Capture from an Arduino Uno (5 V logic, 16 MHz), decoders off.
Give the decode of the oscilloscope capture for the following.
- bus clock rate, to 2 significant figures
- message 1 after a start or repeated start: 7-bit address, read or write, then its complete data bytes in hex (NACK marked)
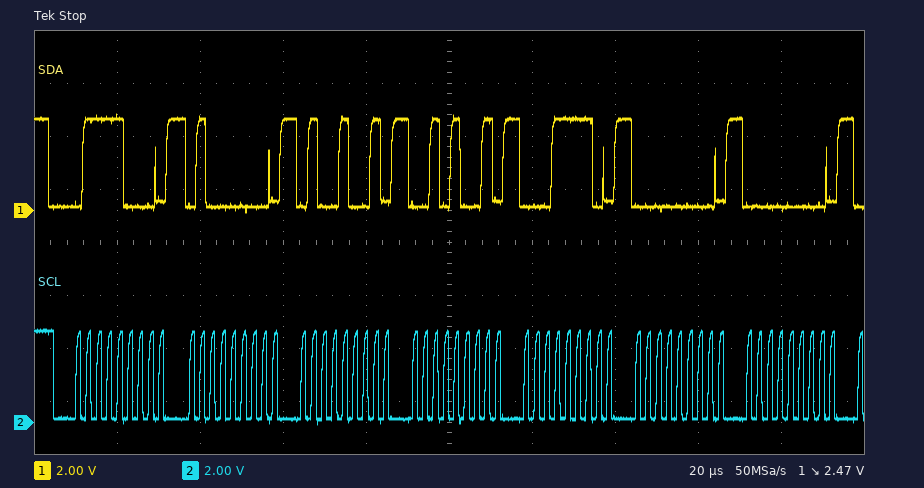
400 kHz
0x3C write: 40 49 29 1E 00 00
